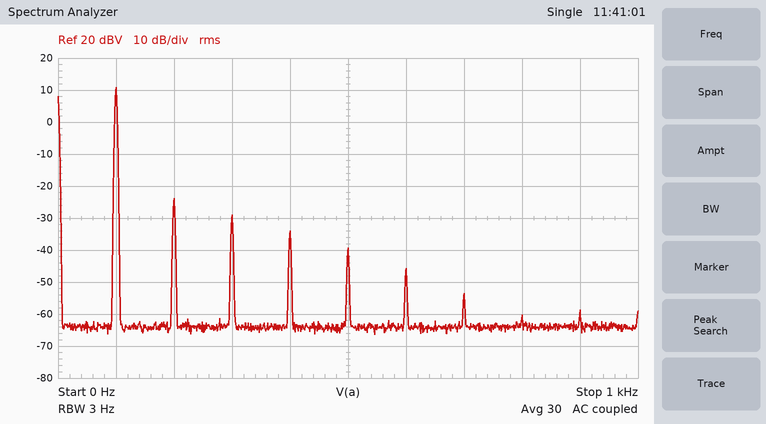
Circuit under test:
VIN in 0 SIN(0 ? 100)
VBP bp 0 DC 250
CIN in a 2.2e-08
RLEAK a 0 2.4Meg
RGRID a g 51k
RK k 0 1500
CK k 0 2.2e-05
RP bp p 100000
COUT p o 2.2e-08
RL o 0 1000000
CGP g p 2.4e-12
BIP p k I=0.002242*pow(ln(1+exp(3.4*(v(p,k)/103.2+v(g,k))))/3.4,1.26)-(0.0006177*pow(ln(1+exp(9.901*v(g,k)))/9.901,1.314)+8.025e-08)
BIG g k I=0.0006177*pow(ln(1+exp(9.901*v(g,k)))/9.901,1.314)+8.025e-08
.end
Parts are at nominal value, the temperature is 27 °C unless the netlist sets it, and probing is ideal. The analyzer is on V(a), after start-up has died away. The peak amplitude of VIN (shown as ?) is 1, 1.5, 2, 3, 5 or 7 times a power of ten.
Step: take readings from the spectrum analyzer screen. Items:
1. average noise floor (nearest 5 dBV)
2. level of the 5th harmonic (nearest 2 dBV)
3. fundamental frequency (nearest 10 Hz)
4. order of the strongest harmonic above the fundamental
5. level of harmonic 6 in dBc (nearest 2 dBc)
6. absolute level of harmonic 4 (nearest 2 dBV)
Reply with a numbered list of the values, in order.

1. -65 dBV
2. -40 dBV
3. 100 Hz
4. 2
5. -56 dBc
6. -34 dBV
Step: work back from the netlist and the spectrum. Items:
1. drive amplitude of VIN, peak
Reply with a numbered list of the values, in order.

1. 5 V
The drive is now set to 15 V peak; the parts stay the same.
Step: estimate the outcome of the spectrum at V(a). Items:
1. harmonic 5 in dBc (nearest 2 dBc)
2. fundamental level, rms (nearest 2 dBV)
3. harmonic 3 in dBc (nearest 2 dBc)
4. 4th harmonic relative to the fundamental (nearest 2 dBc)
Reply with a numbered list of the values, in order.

1. -48 dBc
2. 20 dBV
3. -38 dBc
4. -44 dBc
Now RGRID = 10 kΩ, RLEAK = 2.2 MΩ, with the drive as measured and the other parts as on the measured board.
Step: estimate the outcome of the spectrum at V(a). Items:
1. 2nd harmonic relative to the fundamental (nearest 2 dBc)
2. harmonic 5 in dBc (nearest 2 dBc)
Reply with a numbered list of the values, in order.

1. -32 dBc
2. -44 dBc
